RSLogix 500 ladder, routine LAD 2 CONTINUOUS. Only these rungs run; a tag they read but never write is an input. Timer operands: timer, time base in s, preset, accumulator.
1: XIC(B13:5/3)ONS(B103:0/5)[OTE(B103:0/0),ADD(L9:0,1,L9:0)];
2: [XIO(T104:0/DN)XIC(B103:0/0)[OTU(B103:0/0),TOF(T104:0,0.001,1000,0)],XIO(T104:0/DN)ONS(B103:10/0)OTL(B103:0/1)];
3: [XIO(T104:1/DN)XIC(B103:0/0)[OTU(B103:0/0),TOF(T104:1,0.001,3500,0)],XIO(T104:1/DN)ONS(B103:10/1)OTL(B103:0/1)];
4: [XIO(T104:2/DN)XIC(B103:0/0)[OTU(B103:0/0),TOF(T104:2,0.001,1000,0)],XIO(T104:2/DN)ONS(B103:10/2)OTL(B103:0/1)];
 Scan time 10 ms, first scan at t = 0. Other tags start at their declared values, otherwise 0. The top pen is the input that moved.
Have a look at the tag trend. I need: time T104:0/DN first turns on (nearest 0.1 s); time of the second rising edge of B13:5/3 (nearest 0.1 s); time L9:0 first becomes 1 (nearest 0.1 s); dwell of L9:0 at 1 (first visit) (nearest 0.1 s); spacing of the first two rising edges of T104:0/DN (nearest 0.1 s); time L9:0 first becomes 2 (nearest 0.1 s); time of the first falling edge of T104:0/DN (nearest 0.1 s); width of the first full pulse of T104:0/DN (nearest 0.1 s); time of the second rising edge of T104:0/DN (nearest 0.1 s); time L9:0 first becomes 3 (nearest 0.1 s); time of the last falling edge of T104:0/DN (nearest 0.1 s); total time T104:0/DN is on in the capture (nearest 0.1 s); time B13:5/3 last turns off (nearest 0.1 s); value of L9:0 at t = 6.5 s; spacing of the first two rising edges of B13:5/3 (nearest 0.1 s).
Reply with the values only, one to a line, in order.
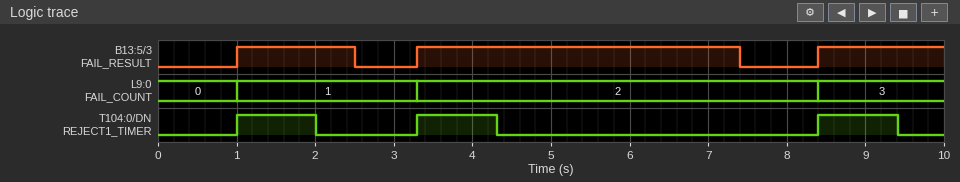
1.0 s
3.3 s
1.0 s
2.3 s
2.3 s
3.3 s
2.0 s
1.0 s
3.3 s
8.4 s
9.4 s
3.0 s
7.4 s
2
2.3 s
